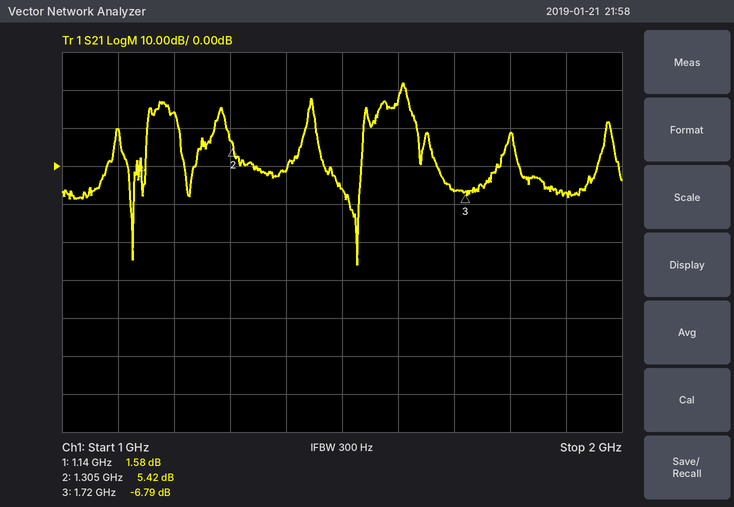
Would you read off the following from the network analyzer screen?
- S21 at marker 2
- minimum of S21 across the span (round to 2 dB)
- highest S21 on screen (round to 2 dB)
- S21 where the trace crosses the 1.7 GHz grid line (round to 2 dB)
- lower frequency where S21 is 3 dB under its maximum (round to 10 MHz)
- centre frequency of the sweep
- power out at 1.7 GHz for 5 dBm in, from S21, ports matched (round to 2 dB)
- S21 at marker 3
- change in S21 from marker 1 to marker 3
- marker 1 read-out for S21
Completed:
5.42 dB
-26 dB
22 dB
-6 dB
1.60 GHz
1.5 GHz
-2 dBm
-6.79 dB
-8.37 dB
1.58 dB
